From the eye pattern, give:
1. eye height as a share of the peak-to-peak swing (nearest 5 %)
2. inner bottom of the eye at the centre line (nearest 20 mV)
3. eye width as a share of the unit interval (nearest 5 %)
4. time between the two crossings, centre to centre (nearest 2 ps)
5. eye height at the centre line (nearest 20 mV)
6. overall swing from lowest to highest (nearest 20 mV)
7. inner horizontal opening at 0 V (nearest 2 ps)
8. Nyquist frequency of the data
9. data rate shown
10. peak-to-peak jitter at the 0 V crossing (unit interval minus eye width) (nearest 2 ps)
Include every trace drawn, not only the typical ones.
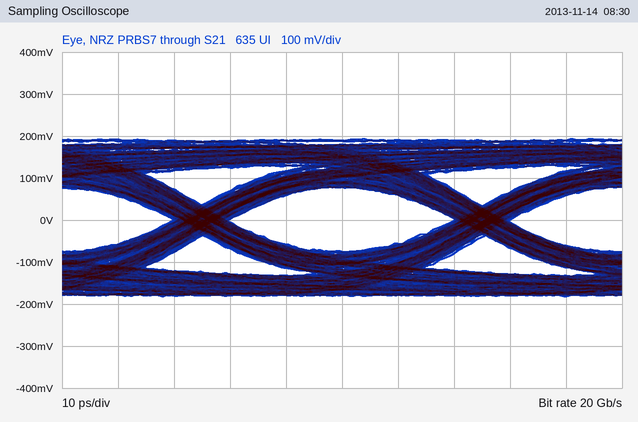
40 %
-80 mV
80 %
50 ps
160 mV
380 mV
40 ps
10 GHz
20 Gb/s
10 ps
